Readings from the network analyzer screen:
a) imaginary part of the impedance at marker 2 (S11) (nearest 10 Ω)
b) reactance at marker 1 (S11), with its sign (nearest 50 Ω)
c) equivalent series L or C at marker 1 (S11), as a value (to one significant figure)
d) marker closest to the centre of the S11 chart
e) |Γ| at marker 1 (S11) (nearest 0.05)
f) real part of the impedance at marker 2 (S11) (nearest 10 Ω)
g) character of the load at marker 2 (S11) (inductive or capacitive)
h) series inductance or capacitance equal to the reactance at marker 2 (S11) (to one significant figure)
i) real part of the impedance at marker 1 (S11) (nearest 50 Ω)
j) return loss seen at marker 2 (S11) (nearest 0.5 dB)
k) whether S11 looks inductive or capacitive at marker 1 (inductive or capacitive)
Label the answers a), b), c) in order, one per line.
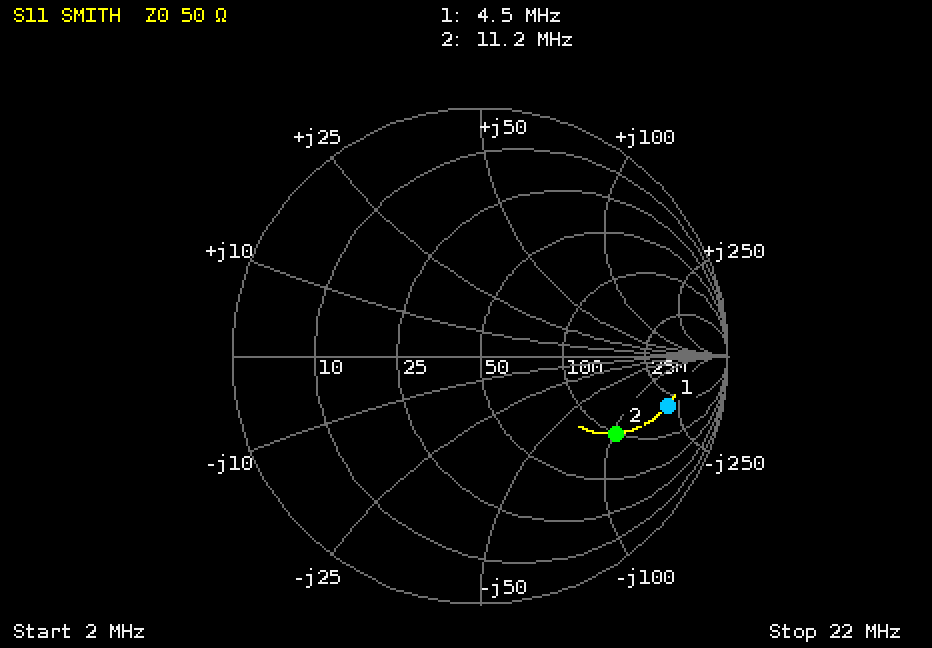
a) -100 Ω
b) -200 Ω
c) 200 pF
d) marker 2
e) 0.80
f) 100 Ω
g) capacitive
h) 100 pF
i) 200 Ω
j) 4.0 dB
k) capacitive
